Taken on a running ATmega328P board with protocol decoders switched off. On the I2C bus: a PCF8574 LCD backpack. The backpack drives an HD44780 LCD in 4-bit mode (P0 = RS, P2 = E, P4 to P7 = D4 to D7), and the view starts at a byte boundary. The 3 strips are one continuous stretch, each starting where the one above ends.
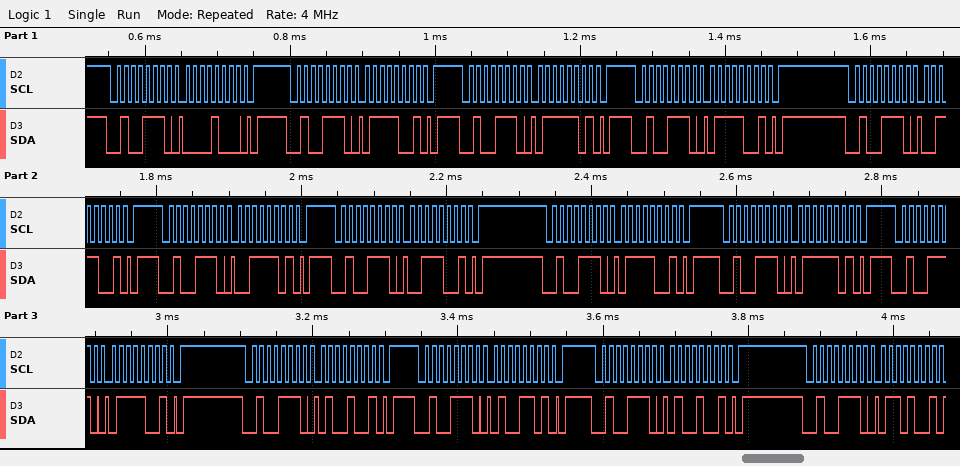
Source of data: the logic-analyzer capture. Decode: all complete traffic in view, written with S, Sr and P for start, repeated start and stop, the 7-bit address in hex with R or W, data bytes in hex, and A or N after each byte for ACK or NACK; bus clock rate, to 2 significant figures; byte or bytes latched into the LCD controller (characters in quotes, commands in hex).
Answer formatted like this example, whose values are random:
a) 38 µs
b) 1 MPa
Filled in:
a) S 27W A 08 A P S 27W A 79 A P S 27W A 7D A P S 27W A 79 A P S 27W A 39 A P S 27W A 3D A P S 27W A 39 A P S 27W A 79 A P S 27W A 7D A P S 27W A 79 A P S 27W A 49 A P S 27W A 4D A P S 27W A 49 A P S 27W A 69 A
b) 100 kHz
c) 's' 't'
